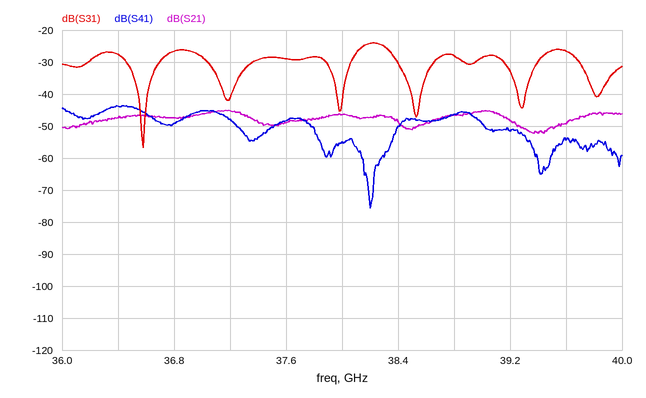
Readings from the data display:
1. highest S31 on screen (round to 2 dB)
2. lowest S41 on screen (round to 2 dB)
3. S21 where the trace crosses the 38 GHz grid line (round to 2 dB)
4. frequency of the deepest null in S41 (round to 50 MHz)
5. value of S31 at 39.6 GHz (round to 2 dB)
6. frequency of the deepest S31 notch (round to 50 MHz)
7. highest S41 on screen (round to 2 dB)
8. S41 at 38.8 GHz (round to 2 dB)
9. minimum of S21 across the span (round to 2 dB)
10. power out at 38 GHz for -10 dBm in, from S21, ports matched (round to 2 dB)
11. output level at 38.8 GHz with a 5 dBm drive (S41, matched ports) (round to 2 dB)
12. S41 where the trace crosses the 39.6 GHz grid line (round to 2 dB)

-24 dB
-76 dB
-46 dB
38.20 GHz
-26 dB
36.60 GHz
-44 dB
-46 dB
-52 dB
-56 dBm
-42 dBm
-54 dB
